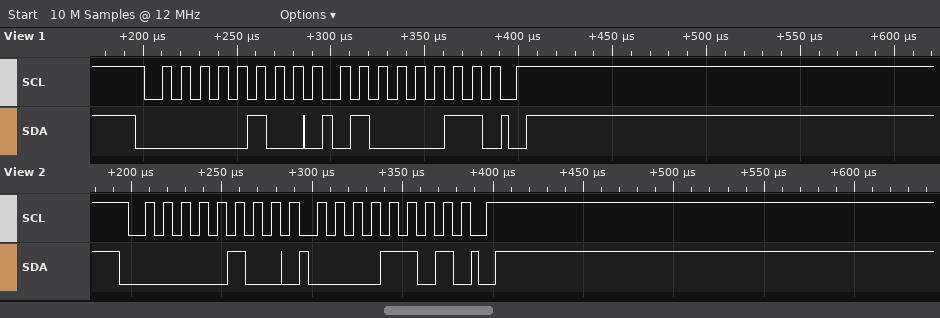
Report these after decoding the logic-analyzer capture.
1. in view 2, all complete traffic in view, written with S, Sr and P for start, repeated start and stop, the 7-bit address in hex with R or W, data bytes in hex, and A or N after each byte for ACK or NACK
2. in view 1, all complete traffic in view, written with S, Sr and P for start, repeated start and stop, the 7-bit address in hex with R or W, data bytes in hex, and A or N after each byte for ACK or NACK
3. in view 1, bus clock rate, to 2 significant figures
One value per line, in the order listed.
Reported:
S 02W A 0D A P
S 02W A 43 A P
100 kHz
